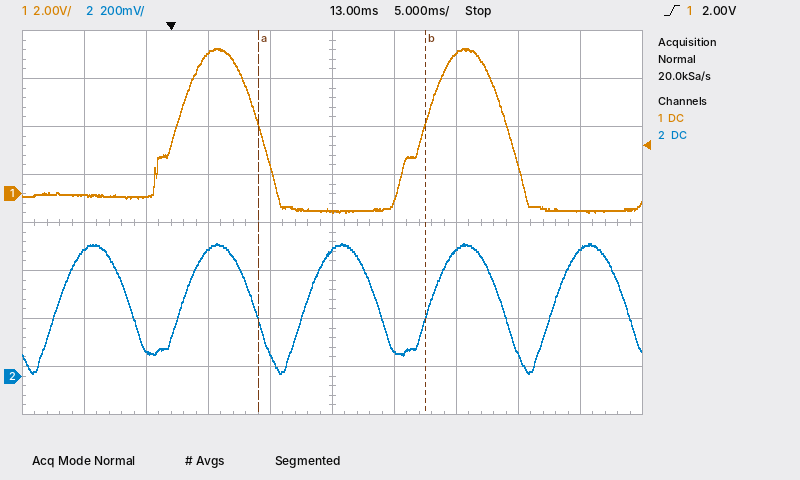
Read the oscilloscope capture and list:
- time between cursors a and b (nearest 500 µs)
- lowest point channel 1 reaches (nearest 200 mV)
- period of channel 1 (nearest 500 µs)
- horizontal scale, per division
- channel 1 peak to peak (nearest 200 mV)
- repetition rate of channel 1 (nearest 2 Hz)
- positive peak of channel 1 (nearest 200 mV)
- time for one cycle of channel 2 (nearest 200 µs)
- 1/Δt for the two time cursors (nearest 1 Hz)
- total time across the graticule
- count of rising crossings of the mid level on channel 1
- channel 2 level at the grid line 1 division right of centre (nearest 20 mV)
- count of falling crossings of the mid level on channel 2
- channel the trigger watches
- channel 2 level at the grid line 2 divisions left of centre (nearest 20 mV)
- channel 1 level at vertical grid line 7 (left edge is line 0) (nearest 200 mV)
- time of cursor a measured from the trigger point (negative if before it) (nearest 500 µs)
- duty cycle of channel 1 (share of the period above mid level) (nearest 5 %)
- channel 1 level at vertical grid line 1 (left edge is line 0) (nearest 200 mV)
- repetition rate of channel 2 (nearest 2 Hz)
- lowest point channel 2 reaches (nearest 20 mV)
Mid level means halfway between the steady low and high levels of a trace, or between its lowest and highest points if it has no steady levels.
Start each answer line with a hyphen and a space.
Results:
- 13.5 ms
- -800 mV
- 20.0 ms
- 5 ms
- 6.8 V
- 50 Hz
- 6.0 V
- 10.0 ms
- 74 Hz
- 50 ms
- 2
- 100 mV
- 5
- channel 1
- 520 mV
- 5.8 V
- +7.0 ms
- 35 %
- 0.0 V
- 100 Hz
- 20 mV
